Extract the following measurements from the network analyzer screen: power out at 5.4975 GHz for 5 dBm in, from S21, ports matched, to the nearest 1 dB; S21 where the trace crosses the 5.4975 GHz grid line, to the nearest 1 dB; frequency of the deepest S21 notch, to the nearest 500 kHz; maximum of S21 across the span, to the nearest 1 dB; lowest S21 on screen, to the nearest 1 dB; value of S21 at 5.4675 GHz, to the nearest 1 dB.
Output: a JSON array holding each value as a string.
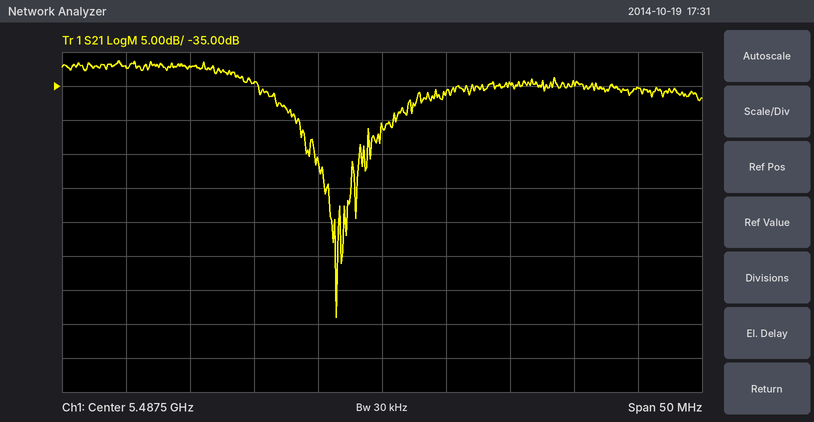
["-30 dBm", "-35 dB", "5.4840 GHz", "-31 dB", "-69 dB", "-32 dB"]
